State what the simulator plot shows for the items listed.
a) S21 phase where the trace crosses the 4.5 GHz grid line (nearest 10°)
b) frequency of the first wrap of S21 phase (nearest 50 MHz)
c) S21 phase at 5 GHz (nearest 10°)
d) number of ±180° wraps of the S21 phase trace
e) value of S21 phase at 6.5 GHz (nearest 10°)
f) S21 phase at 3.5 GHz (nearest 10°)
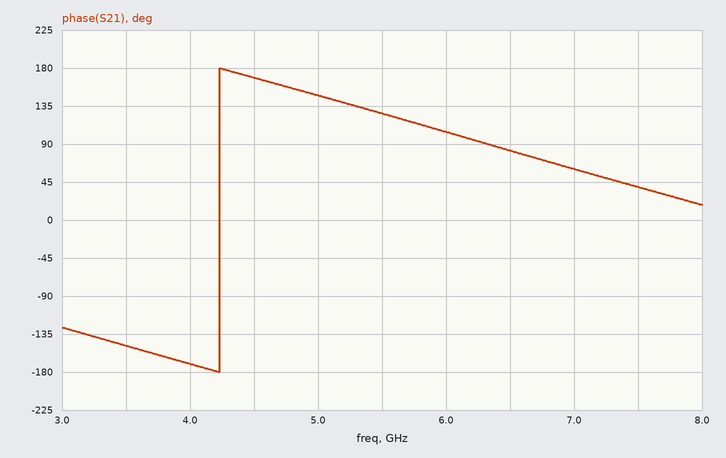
170°
4.25 GHz
150°
1
80°
-150°
